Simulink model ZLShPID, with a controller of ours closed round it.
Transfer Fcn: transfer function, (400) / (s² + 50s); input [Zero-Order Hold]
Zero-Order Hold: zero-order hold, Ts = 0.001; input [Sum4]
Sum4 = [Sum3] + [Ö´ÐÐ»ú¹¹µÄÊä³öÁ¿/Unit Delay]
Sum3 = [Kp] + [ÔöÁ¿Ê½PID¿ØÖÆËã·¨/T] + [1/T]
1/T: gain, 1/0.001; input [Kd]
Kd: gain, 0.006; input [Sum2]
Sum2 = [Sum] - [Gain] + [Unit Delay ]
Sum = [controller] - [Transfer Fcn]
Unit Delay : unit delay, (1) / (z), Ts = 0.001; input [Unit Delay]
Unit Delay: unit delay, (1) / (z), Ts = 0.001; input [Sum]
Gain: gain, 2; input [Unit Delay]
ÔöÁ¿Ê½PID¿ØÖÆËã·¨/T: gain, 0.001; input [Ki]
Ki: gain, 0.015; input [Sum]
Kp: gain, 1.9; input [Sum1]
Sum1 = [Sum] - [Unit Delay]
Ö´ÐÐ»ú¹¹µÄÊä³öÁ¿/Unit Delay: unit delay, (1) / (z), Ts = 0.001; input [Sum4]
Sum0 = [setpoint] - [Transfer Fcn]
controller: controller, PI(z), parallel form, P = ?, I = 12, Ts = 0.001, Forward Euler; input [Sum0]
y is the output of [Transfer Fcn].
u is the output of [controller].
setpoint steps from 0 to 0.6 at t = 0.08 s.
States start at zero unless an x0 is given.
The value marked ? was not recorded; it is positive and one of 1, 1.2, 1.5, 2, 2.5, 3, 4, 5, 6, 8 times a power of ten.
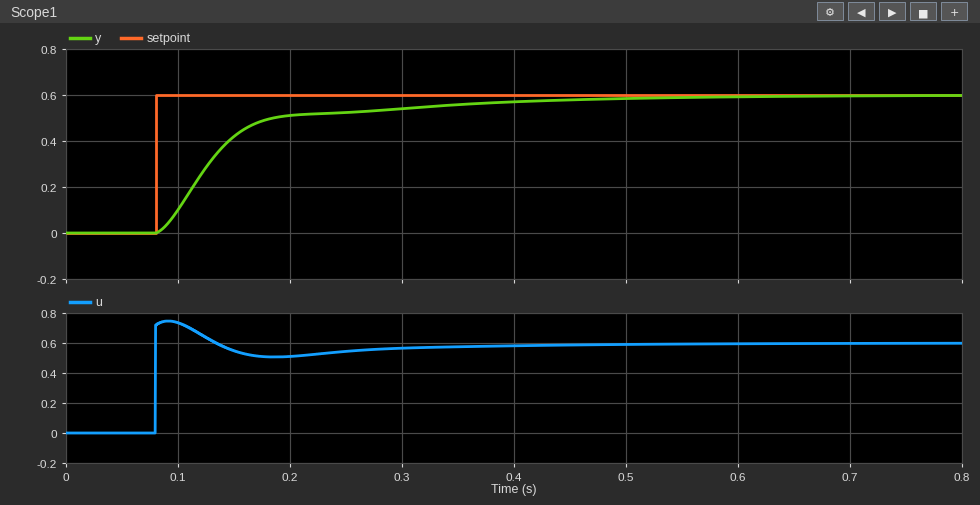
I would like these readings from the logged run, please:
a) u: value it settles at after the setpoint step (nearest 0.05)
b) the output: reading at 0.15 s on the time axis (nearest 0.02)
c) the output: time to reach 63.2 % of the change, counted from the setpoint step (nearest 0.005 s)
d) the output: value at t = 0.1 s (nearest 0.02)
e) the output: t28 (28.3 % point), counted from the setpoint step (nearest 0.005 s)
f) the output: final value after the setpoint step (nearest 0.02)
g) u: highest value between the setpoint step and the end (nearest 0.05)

0.60
0.42
0.060 s
0.10
0.030 s
0.60
0.75
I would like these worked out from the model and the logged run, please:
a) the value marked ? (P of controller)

1.2
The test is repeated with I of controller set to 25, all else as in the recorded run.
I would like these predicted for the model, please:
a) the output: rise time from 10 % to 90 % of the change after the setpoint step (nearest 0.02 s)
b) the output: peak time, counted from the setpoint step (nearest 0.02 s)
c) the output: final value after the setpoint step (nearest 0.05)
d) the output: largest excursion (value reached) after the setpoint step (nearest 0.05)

0.06 s
0.12 s
0.60
0.65
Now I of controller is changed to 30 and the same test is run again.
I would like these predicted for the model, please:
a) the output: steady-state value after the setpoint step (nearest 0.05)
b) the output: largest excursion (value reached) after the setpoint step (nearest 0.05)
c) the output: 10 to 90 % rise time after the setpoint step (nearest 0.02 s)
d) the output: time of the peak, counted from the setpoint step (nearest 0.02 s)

0.60
0.70
0.06 s
0.12 s
